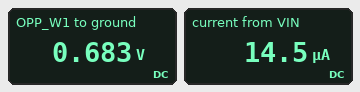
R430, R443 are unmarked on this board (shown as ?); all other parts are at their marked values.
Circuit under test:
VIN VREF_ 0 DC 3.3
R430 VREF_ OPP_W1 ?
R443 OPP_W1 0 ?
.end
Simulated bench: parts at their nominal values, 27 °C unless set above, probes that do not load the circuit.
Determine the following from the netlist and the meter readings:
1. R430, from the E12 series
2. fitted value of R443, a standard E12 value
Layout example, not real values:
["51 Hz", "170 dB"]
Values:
["180 kΩ", "47 kΩ"]
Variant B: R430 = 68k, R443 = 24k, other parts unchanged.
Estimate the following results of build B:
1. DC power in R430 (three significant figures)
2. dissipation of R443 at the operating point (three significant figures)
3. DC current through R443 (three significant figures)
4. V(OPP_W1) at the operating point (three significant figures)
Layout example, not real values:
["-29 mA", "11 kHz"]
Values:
["87.5 µW", "30.9 µW", "35.9 µA", "861 mV"]
